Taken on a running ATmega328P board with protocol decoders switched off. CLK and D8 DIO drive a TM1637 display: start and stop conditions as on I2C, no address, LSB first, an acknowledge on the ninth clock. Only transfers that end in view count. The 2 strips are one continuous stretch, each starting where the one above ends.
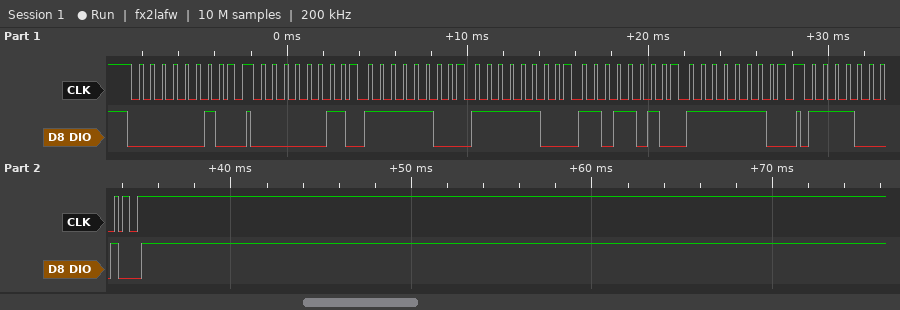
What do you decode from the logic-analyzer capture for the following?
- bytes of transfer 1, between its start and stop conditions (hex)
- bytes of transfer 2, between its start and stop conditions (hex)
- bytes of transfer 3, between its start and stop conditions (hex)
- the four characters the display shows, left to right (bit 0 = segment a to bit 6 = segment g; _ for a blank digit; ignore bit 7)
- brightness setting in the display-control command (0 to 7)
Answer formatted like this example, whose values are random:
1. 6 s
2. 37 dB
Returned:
1. 40
2. C0 3F 3F 5B 7F
3. 8F
4. 0028
5. 7
